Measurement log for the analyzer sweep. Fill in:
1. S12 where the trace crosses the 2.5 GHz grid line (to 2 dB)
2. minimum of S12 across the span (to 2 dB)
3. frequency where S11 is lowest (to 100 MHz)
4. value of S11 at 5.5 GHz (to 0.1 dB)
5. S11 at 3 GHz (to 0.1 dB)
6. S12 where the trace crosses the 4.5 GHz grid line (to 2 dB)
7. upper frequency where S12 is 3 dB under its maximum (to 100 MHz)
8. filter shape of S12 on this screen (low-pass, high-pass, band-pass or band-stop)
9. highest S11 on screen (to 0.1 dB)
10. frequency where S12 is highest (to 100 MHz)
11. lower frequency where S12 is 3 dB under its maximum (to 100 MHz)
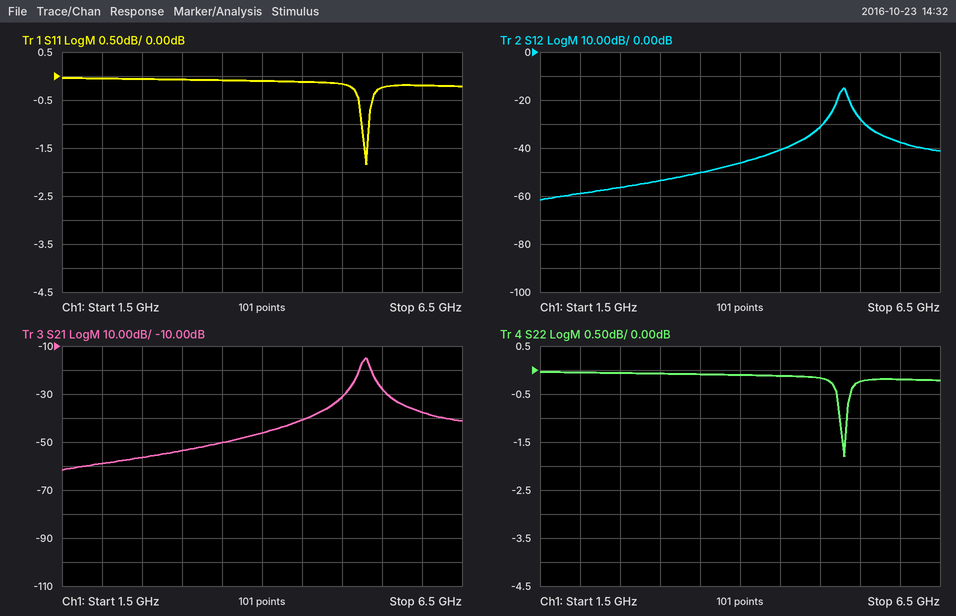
-56 dB
-62 dB
5.3 GHz
-0.2 dB
-0.1 dB
-40 dB
5.3 GHz
band-pass
0.0 dB
5.3 GHz
5.2 GHz
